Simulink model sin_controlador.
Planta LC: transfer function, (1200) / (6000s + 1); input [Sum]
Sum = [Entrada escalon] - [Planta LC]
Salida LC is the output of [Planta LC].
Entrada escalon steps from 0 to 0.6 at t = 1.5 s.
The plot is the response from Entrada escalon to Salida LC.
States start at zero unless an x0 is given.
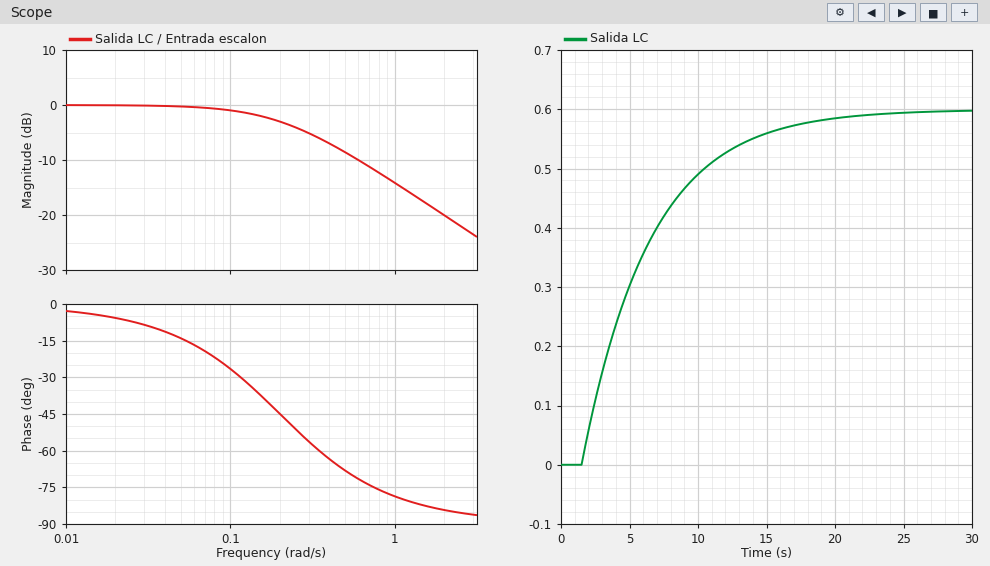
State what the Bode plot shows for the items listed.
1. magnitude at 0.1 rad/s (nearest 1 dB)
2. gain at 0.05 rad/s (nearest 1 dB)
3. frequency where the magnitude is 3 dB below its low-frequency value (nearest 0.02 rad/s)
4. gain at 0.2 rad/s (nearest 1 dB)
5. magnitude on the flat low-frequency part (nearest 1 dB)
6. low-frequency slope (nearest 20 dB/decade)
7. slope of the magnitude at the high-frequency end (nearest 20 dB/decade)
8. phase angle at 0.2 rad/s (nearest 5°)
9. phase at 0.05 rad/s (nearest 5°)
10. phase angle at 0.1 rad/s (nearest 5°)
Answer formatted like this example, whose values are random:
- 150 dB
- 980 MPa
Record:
- -1 dB
- 0 dB
- 0.20 rad/s
- -3 dB
- 0 dB
- 0 dB/decade
- -20 dB/decade
- -45°
- -15°
- -25°
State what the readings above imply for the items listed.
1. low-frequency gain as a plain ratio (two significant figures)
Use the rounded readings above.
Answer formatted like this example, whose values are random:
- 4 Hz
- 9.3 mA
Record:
- 1.0
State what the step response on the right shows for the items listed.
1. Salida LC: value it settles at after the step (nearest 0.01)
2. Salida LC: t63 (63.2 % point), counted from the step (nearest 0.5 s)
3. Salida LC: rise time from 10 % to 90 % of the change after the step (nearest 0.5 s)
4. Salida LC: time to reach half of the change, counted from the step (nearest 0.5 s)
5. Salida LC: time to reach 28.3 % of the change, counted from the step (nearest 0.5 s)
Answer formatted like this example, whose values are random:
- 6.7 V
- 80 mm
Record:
- 0.60
- 5.0 s
- 11.0 s
- 3.5 s
- 1.5 s
